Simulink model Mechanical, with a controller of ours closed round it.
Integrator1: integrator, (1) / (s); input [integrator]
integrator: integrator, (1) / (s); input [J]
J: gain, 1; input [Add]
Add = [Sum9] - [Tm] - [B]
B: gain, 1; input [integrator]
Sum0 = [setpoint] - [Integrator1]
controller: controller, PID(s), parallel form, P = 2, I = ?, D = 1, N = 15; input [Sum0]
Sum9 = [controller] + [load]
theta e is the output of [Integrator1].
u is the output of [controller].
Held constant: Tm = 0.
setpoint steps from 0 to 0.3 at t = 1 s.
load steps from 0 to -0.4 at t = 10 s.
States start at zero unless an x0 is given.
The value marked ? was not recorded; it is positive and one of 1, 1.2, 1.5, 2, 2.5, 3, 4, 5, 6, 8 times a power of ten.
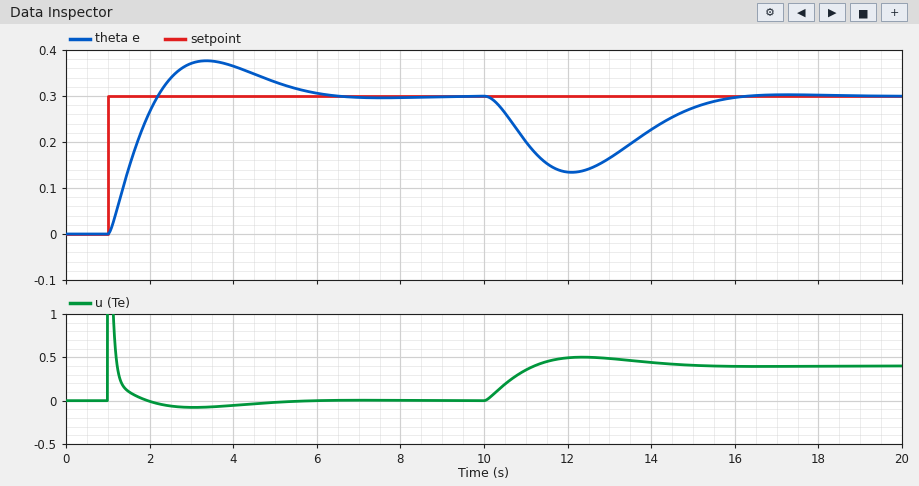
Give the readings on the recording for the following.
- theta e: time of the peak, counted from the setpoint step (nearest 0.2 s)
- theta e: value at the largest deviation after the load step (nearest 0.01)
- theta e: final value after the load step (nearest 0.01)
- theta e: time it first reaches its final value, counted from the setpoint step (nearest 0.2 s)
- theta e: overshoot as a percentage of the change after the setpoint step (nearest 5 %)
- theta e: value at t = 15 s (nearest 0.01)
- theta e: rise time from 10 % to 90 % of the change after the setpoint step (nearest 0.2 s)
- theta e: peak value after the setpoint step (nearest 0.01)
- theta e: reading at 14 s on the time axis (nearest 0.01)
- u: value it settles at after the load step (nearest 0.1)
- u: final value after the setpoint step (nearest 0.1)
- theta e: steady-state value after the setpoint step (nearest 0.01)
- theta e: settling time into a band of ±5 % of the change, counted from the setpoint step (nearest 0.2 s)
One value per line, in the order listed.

2.4 s
0.13
0.30
1.2 s
25 %
0.27
0.8 s
0.38
0.23
0.4
0.0
0.30
4.6 s
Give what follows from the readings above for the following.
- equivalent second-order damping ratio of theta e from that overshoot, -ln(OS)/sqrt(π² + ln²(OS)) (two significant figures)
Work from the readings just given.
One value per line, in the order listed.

0.40
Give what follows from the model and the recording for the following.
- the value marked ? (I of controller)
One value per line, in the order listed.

0.8
